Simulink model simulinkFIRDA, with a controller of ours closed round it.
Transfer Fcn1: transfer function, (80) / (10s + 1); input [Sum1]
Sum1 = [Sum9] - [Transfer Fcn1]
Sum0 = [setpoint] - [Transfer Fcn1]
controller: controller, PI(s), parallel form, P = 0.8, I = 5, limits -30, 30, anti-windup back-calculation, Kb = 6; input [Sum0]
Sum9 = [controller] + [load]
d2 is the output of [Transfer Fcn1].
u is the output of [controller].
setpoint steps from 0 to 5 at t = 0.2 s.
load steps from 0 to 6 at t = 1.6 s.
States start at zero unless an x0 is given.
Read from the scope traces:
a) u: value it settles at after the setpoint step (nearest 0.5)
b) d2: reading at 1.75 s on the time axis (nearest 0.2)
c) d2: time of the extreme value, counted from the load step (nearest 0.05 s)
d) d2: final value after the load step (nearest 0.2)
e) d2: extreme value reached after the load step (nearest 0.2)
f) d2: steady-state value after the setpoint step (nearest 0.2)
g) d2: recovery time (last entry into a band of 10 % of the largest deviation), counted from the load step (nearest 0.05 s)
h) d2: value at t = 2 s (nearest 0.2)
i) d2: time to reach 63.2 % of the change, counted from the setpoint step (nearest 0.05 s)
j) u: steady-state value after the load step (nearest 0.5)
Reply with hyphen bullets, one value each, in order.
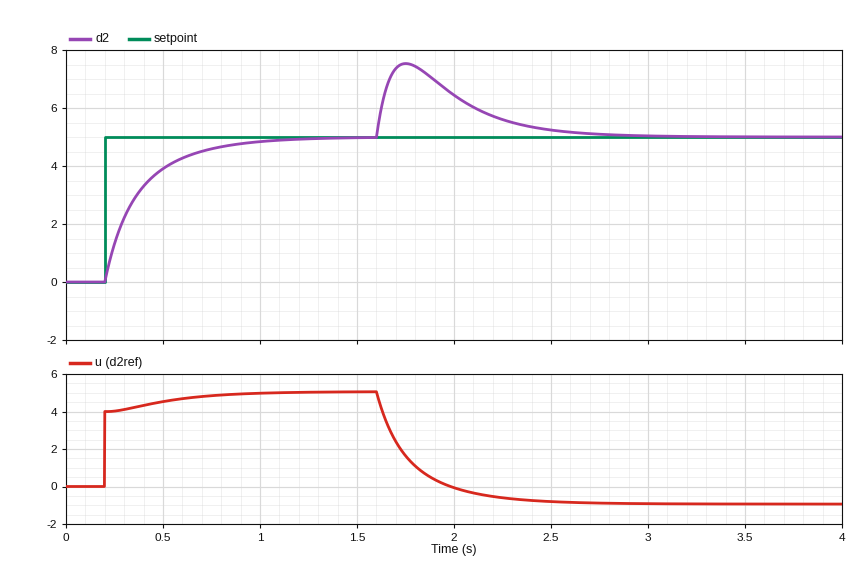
- 5.0
- 7.6
- 0.15 s
- 5.0
- 7.6
- 5.0
- 0.90 s
- 6.4
- 0.20 s
- -1.0
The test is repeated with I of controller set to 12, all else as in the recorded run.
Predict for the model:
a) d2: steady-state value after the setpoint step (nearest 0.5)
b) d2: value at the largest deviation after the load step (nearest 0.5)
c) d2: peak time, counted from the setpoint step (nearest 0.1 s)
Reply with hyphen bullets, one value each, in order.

- 5.0
- 7.0
- 0.4 s
